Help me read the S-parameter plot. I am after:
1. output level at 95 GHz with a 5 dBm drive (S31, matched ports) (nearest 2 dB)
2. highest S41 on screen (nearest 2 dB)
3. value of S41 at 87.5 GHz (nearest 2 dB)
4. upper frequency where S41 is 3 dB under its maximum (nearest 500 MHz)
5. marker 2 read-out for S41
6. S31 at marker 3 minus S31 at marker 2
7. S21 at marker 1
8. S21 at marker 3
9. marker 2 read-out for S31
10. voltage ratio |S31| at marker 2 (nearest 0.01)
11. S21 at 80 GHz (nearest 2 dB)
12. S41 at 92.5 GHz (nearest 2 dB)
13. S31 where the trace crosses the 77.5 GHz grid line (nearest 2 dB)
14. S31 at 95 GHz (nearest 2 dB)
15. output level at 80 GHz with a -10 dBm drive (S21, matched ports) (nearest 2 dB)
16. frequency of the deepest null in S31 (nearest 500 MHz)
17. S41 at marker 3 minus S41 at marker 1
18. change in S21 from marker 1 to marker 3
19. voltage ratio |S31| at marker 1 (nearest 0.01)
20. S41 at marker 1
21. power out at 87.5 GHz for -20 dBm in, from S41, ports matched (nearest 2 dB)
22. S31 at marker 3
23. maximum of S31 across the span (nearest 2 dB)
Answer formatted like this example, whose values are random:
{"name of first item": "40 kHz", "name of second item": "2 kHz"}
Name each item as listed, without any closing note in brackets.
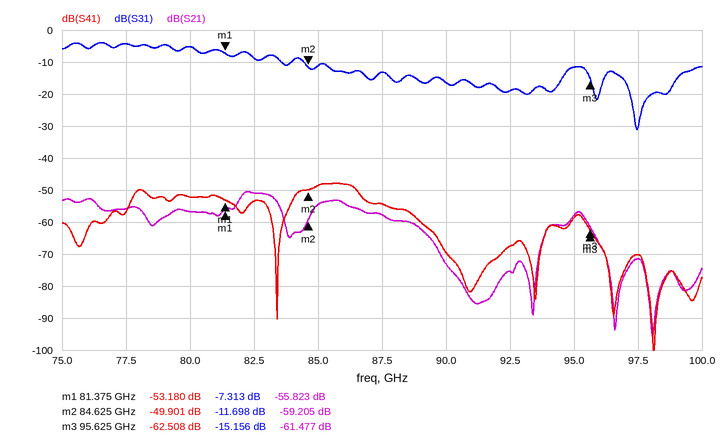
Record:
{"output level at 95 GHz with a 5 dBm drive (S31, matched ports)": "-6 dBm", "highest S41 on screen": "-48 dB", "value of S41 at 87.5 GHz": "-54 dB", "upper frequency where S41 is 3 dB under its maximum": "86.5 GHz", "marker 2 read-out for S41": "-49.901 dB", "S31 at marker 3 minus S31 at marker 2": "-3.458 dB", "S21 at marker 1": "-55.823 dB", "S21 at marker 3": "-61.477 dB", "marker 2 read-out for S31": "-11.698 dB", "voltage ratio |S31| at marker 2": "0.26", "S21 at 80 GHz": "-56 dB", "S41 at 92.5 GHz": "-68 dB", "S31 where the trace crosses the 77.5 GHz grid line": "-4 dB", "S31 at 95 GHz": "-12 dB", "output level at 80 GHz with a -10 dBm drive (S21, matched ports)": "-66 dBm", "frequency of the deepest null in S31": "97.5 GHz", "S41 at marker 3 minus S41 at marker 1": "-9.328 dB", "change in S21 from marker 1 to marker 3": "-5.654 dB", "voltage ratio |S31| at marker 1": "0.43", "S41 at marker 1": "-53.180 dB", "power out at 87.5 GHz for -20 dBm in, from S41, ports matched": "-74 dBm", "S31 at marker 3": "-15.156 dB", "maximum of S31 across the span": "-4 dB"}
